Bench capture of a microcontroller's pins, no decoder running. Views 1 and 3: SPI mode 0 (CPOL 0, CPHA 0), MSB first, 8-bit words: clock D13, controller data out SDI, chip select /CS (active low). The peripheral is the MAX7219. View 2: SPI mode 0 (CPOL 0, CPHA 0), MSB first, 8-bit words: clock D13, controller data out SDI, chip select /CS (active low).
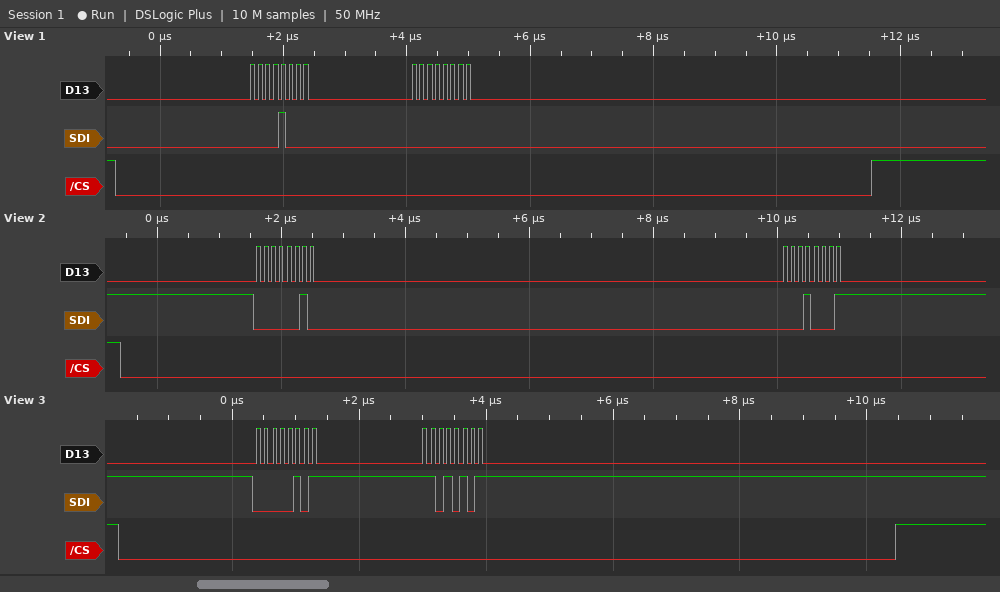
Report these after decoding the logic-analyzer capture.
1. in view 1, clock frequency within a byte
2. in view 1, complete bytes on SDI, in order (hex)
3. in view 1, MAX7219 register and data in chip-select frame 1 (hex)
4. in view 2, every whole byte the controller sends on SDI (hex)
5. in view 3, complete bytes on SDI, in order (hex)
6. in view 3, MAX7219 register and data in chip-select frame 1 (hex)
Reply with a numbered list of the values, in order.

1. 8 MHz
2. 08 00
3. register 0x8, data 0x00
4. 0x02 0x11
5. 05 D5
6. register 0x5, data 0xD5
